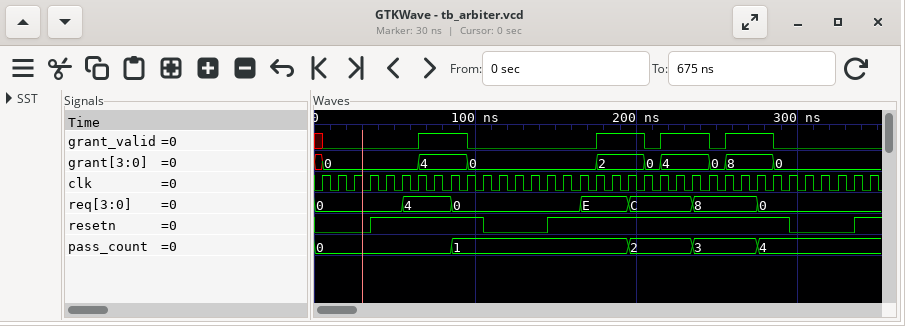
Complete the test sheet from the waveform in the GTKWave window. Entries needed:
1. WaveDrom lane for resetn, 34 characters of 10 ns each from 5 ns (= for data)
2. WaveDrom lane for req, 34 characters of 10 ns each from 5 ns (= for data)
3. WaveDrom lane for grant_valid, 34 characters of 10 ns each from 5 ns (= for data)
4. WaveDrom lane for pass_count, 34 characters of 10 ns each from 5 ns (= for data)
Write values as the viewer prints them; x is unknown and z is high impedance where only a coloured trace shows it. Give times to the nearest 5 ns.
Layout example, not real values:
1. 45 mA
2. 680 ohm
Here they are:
1. {name: 'resetn', wave: '0..1......0...1..............0...1'}
2. {name: 'req', wave: '=....=..=.......=..=...=...=......', data: '0 4 0 E C 8 0'}
3. {name: 'grant_valid', wave: '0.....1..0.......1..01..01..0.....'}
4. {name: 'pass_count', wave: '=.......=..........=...=...=......', data: '0 1 2 3 4'}
